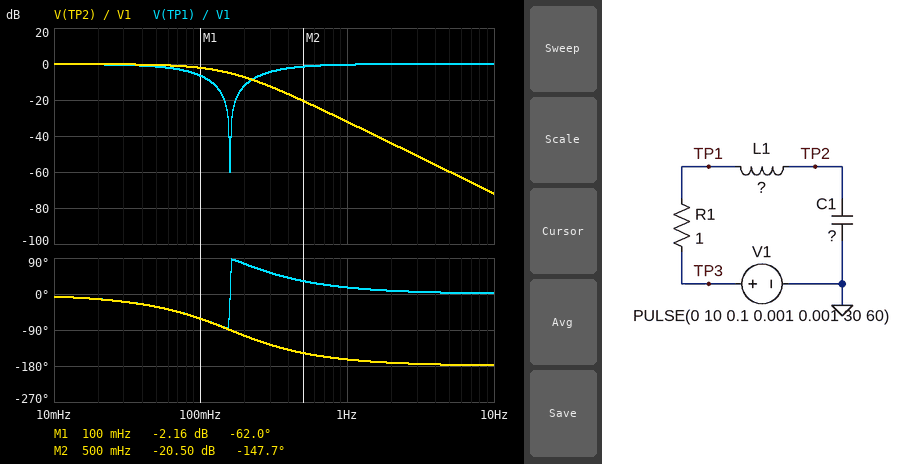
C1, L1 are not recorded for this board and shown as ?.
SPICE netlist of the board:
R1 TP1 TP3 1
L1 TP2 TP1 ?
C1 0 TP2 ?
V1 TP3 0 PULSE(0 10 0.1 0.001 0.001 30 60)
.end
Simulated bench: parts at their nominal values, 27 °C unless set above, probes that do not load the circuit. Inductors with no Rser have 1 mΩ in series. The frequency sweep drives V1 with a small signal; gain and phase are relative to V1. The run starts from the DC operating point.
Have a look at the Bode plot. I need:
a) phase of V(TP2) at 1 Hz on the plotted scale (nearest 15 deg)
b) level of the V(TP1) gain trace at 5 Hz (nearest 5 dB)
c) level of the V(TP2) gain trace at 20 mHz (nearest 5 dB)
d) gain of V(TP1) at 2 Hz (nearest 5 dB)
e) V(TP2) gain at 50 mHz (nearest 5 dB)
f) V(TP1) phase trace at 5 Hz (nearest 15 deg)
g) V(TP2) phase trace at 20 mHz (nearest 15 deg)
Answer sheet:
-165 deg
0 dB
0 dB
0 dB
0 dB
0 deg
-15 deg
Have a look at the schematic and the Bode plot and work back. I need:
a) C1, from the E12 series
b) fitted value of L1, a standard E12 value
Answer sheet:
1.8 F
560 mH
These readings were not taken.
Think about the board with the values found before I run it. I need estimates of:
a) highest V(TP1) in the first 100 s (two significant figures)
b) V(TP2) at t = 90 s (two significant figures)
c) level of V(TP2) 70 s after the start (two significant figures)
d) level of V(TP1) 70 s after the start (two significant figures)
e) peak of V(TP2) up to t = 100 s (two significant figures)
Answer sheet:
10 V
10 V
10 V
10 V
10 V
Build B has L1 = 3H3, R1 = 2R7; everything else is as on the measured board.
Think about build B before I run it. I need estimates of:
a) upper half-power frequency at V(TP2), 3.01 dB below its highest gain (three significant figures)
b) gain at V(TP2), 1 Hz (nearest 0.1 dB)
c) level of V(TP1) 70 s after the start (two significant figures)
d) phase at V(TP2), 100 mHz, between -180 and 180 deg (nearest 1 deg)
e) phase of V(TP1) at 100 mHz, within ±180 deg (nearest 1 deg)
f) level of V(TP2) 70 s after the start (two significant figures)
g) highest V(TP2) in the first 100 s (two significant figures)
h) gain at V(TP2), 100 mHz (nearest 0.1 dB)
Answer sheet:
42.2 mHz
-47.4 dB
8.6 V
-114 deg
66 deg
9.1 V
10 V
-10.5 dB
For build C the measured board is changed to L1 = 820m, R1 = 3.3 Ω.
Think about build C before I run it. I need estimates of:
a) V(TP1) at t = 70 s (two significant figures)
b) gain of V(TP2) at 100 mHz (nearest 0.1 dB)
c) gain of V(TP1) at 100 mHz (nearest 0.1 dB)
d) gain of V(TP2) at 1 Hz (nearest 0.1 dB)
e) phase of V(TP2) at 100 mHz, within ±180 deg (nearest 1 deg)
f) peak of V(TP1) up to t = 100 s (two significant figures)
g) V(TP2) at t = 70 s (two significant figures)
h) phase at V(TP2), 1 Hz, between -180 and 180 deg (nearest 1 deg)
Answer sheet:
8.1 V
-11.5 dB
-19.1 dB
-36.7 dB
-84 deg
10 V
8.2 V
-147 deg
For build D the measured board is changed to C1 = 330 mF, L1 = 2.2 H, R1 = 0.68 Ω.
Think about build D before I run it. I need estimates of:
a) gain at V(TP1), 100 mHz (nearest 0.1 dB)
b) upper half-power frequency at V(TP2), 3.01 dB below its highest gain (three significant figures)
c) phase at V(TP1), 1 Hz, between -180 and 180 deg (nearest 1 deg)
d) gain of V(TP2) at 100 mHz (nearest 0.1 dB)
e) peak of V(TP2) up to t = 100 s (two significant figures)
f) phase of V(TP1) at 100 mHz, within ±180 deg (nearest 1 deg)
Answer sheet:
-0.2 dB
207 mHz
3 deg
2.8 dB
17 V
-11 deg
